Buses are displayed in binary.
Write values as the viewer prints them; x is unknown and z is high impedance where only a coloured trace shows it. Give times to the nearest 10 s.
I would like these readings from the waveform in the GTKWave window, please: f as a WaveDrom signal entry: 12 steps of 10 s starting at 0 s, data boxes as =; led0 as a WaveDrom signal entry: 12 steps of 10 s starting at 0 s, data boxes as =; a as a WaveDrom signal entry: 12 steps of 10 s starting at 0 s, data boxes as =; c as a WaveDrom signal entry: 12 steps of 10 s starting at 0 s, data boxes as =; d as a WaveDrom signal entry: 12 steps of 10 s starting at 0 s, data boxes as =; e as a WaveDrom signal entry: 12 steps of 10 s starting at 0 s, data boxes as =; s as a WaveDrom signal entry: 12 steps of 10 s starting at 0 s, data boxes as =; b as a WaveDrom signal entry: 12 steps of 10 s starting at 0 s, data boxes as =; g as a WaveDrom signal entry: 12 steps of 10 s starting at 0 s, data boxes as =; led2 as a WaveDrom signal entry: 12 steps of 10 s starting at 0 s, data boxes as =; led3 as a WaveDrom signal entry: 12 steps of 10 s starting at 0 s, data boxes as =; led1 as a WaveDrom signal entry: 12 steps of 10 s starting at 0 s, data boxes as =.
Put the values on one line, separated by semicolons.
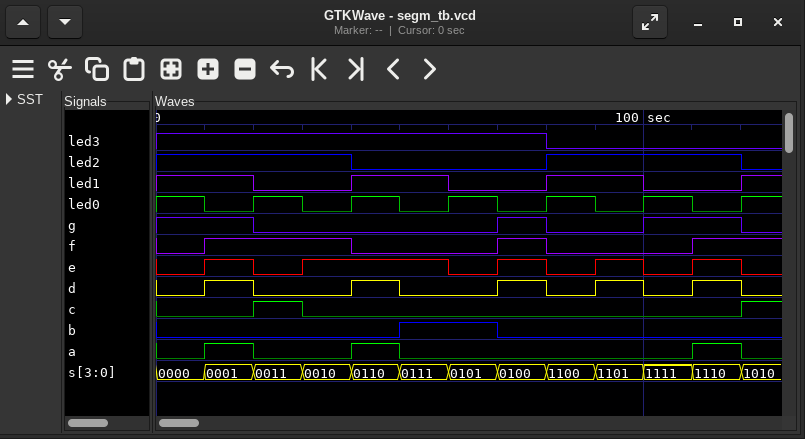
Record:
{name: 'f', wave: '01..0..10..1'}; {name: 'led0', wave: '101010101010'}; {name: 'a', wave: '010.10.....1'}; {name: 'c', wave: '0.10........'}; {name: 'd', wave: '010.10.10101'}; {name: 'e', wave: '0101..010101'}; {name: 's', wave: '============', data: '0000 0001 0011 0010 0110 0111 0101 0100 1100 1101 1111 1110'}; {name: 'b', wave: '0....1.0....'}; {name: 'g', wave: '1.0....10.1.'}; {name: 'led2', wave: '1...0...1...'}; {name: 'led3', wave: '1.......0...'}; {name: 'led1', wave: '1.0.1.0.1.0.'}
